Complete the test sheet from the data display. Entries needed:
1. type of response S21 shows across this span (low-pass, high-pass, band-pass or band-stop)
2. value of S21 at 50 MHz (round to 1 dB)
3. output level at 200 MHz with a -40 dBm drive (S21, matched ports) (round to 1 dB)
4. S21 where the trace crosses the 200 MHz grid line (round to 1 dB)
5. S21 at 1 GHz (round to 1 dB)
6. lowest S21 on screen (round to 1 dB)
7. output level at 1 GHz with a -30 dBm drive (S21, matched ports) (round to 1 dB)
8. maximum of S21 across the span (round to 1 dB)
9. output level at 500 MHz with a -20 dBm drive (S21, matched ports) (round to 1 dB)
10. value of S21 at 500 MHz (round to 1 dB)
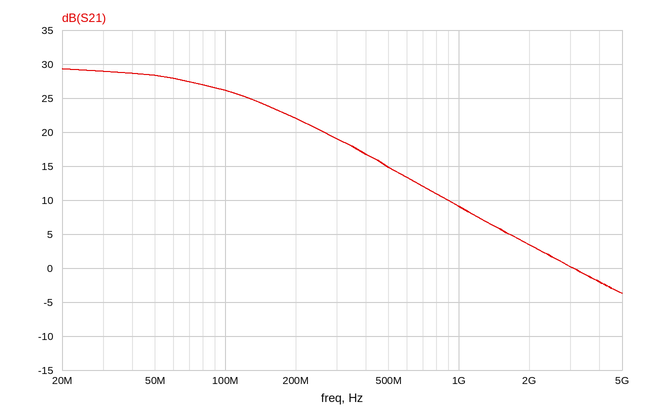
low-pass
28 dB
-18 dBm
22 dB
9 dB
-4 dB
-21 dBm
29 dB
-5 dBm
15 dB
